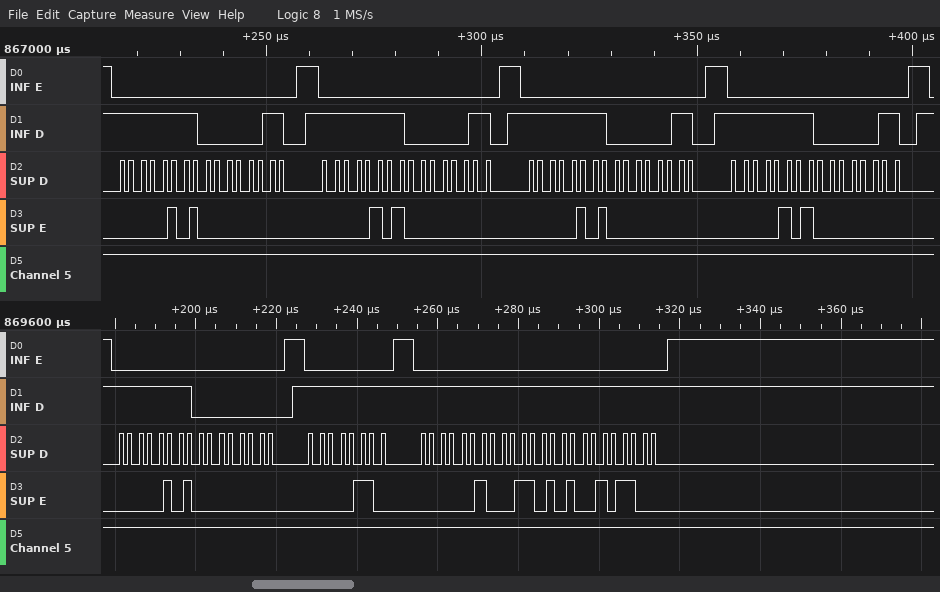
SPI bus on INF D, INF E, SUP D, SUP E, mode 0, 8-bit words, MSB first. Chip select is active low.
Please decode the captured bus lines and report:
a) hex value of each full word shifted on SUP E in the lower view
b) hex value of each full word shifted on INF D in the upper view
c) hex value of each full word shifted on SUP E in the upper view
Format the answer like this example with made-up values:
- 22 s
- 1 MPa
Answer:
- 05, 00, 06, 02, 35, 2C
- FF, 03, FF, 03, FF, 03, FF, 03
- 05, 00, 05, 00, 05, 00, 05, 00
